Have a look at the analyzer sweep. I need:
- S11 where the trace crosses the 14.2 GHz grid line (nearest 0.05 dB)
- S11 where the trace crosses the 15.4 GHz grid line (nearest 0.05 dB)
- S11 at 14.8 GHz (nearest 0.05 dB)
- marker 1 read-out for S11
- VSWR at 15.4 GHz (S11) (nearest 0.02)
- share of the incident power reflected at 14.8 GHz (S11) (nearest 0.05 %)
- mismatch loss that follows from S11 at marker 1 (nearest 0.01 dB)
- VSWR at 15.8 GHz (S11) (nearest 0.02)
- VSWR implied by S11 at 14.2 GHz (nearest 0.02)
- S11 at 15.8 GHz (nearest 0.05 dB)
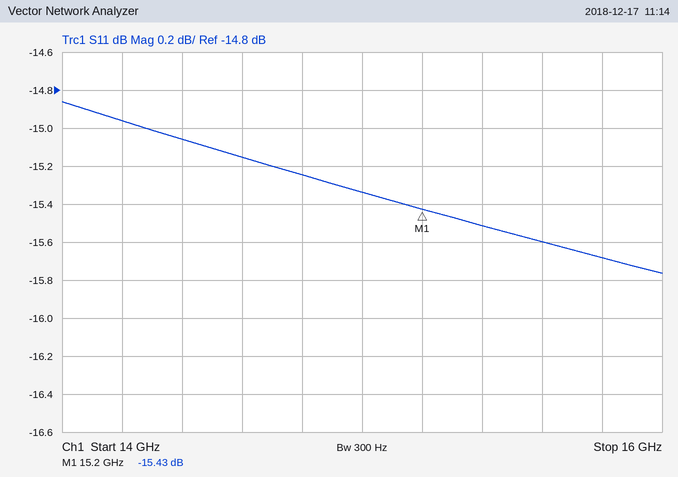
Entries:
-14.95 dB
-15.50 dB
-15.25 dB
-15.43 dB
1.40
3.00 %
0.13 dB
1.40
1.44
-15.70 dB
